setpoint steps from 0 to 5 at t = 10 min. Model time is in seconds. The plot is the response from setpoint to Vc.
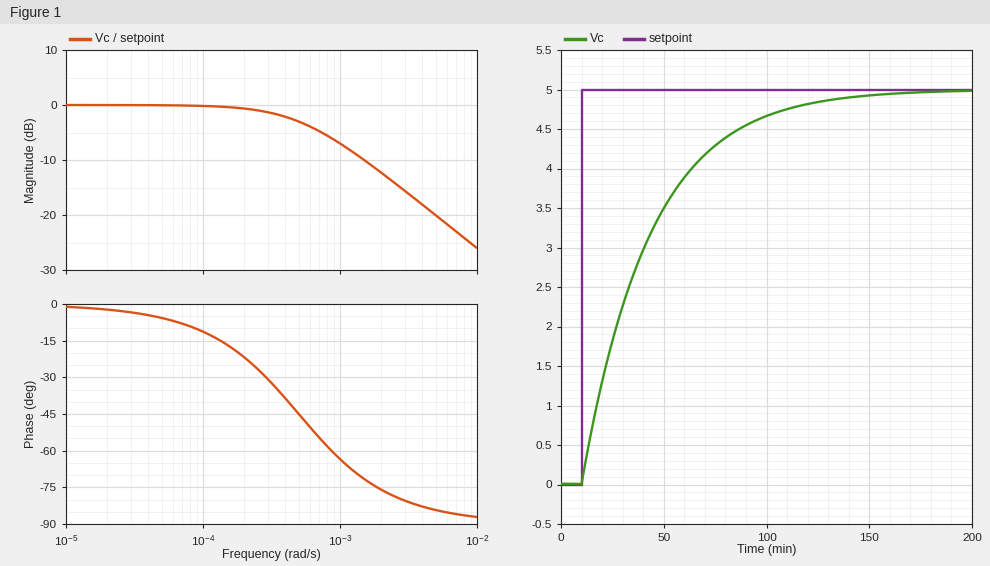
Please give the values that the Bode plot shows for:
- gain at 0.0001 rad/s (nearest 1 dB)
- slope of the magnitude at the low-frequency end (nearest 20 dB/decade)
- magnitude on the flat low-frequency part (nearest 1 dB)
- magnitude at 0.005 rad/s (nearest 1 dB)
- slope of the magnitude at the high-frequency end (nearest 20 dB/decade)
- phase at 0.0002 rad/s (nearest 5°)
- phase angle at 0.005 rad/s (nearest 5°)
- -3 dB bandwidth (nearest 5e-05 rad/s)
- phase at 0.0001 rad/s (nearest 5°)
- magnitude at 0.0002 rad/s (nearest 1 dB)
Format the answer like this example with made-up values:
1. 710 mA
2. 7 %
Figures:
1. 0 dB
2. 0 dB/decade
3. 0 dB
4. -20 dB
5. -20 dB/decade
6. -20°
7. -85°
8. 0.00050 rad/s
9. -10°
10. -1 dB
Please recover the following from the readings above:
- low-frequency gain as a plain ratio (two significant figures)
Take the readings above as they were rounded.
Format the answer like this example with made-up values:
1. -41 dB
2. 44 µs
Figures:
1. 1.0
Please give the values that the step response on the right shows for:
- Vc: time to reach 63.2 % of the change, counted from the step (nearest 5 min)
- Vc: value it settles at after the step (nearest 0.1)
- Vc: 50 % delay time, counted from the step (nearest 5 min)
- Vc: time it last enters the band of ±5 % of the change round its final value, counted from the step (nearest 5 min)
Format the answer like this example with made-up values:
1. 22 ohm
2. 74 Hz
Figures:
1. 35 min
2. 5.0
3. 25 min
4. 100 min
